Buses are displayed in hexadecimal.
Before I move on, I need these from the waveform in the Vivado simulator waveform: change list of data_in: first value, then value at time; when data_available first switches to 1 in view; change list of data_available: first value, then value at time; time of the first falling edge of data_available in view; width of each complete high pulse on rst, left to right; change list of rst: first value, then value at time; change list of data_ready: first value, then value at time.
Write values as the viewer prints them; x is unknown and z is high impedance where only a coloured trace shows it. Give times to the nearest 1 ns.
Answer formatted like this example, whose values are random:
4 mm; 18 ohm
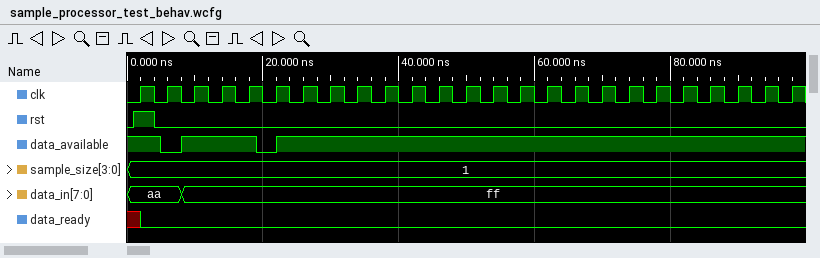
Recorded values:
aa, ff at 8 ns; 8 ns; 1, 0 at 5 ns, 1 at 8 ns, 0 at 19 ns, 1 at 22 ns; 5 ns; 3 ns; 0, 1 at 1 ns, 0 at 4 ns; x, 0 at 2 ns
